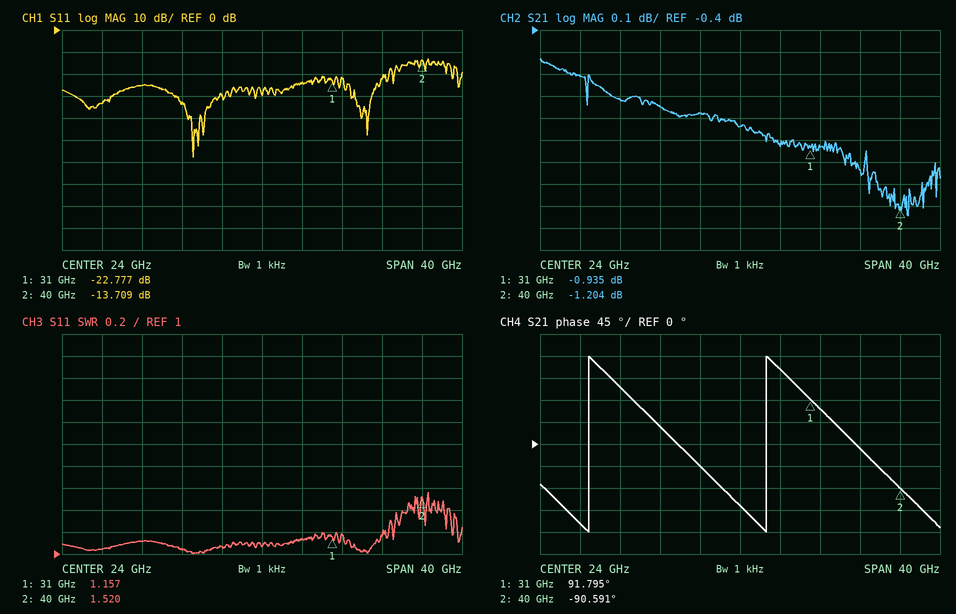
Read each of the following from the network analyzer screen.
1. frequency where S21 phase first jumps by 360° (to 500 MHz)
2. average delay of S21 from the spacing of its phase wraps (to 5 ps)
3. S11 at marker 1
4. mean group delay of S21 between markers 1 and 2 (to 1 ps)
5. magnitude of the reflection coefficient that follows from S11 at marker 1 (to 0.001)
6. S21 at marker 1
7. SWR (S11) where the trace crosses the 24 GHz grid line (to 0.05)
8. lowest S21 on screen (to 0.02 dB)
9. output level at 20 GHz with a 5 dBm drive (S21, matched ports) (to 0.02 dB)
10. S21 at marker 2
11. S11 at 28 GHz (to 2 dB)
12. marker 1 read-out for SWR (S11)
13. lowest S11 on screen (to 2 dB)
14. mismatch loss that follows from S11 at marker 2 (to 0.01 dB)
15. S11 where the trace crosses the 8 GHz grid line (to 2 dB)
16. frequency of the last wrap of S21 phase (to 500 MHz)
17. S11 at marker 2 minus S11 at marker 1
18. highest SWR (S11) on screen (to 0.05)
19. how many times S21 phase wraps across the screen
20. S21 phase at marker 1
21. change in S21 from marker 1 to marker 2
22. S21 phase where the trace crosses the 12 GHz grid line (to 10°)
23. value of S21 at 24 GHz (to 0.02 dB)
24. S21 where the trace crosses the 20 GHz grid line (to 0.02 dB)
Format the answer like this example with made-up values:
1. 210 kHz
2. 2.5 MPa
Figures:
1. 9.0 GHz
2. 55 ps
3. -22.777 dB
4. 56 ps
5. 0.073
6. -0.935 dB
7. 1.05
8. -1.24 dB
9. 4.22 dBm
10. -1.204 dB
11. -24 dB
12. 1.157
13. -58 dB
14. 0.19 dB
15. -34 dB
16. 26.5 GHz
17. 9.068 dB
18. 1.55
19. 2
20. 91.795°
21. -0.269 dB
22. 120°
23. -0.84 dB
24. -0.78 dB
